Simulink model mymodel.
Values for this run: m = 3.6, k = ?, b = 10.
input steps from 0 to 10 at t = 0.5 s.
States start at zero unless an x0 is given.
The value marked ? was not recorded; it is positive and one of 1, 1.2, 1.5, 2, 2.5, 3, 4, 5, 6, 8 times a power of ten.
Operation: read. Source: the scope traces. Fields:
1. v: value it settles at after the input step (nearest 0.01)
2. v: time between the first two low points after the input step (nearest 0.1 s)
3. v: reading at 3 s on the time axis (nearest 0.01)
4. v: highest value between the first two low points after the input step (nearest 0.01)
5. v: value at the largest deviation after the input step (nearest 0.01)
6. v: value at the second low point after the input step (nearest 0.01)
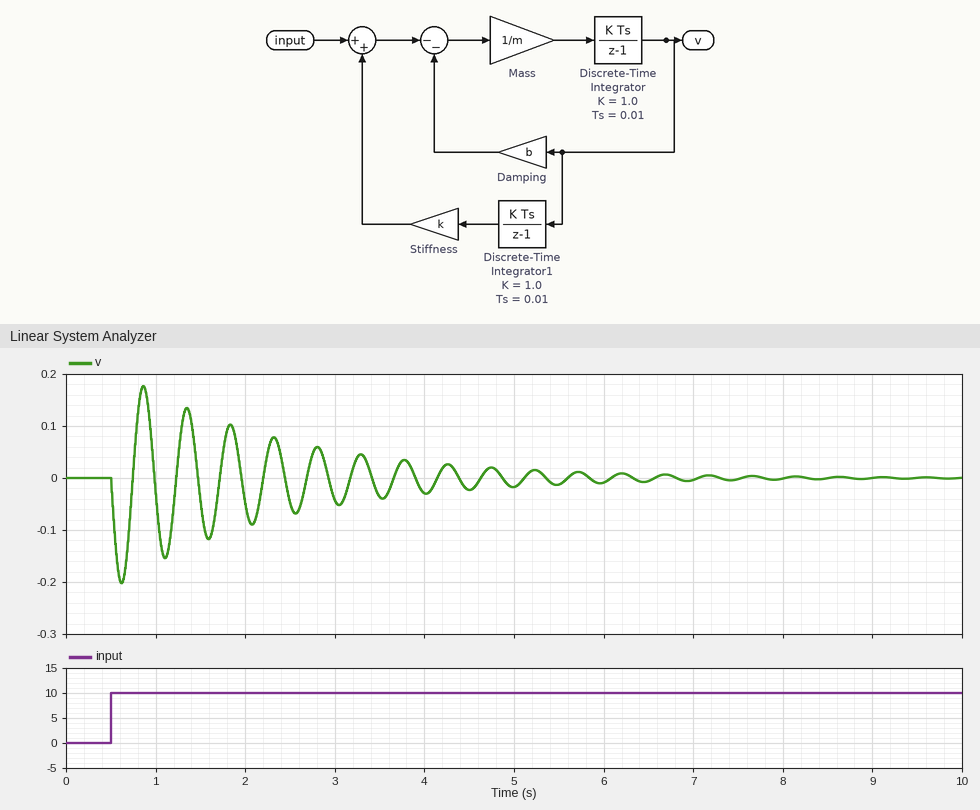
0.00
0.5 s
-0.04
0.18
-0.20
-0.15
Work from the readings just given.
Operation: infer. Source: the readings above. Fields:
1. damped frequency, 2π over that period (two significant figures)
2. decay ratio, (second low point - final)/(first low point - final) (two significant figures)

13 rad/s
0.75
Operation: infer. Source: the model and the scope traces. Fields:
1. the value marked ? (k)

600
